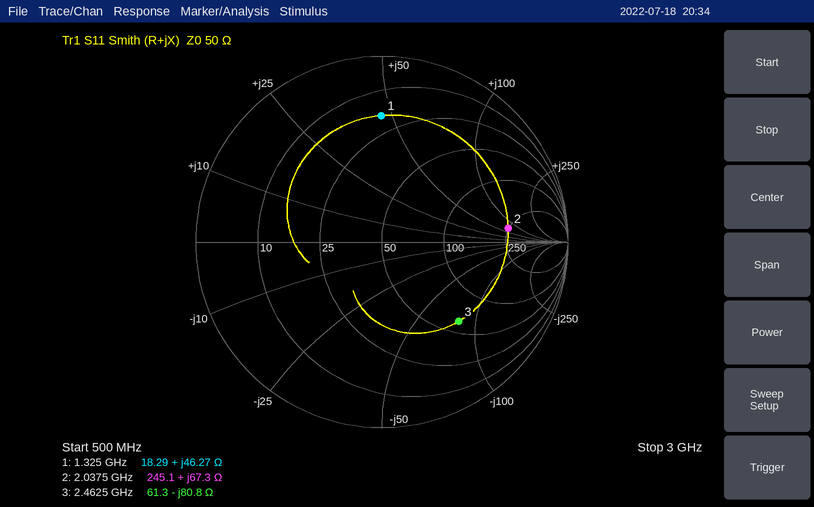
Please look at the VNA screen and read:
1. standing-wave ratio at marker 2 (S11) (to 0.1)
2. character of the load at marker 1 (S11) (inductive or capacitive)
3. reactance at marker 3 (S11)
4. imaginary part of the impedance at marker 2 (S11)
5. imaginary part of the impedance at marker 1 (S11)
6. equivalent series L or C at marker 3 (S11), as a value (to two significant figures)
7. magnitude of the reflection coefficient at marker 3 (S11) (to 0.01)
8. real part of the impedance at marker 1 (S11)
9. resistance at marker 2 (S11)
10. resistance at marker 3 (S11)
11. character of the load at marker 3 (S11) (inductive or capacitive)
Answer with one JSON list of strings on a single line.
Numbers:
["5.3", "inductive", "-80.8 Ω", "+67.3 Ω", "+46.27 Ω", "800 fF", "0.59", "18.29 Ω", "245.1 Ω", "61.3 Ω", "capacitive"]
